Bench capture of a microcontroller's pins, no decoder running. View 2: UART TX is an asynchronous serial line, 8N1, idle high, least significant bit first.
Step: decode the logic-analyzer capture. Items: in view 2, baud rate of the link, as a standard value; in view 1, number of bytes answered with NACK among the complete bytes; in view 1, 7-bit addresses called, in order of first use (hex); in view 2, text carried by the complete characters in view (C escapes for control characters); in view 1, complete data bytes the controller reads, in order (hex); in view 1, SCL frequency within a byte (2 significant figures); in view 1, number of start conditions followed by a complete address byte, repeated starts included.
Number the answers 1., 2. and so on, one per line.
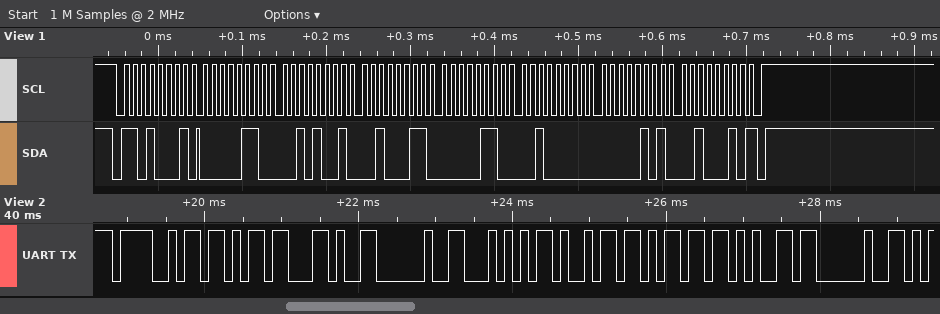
1. 9600 baud
2. 1
3. 0x68
4. "Ok, Time "
5. 06 29 23 06 20 05 22
6. 100 kHz
7. 1
